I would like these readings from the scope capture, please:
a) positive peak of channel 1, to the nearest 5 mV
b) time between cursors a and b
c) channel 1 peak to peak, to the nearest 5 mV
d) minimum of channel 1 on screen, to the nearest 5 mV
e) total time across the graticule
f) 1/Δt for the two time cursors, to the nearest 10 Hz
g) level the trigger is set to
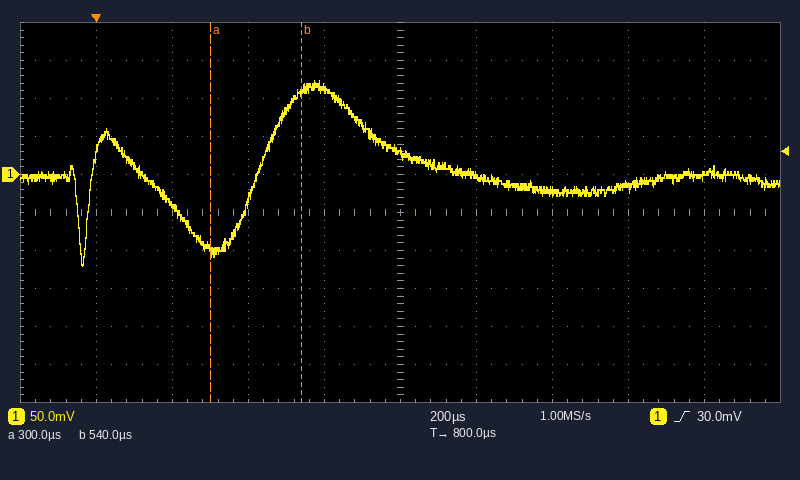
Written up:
125 mV
240 µs
245 mV
-120 mV
2 ms
4.17 kHz
30.0 mV
